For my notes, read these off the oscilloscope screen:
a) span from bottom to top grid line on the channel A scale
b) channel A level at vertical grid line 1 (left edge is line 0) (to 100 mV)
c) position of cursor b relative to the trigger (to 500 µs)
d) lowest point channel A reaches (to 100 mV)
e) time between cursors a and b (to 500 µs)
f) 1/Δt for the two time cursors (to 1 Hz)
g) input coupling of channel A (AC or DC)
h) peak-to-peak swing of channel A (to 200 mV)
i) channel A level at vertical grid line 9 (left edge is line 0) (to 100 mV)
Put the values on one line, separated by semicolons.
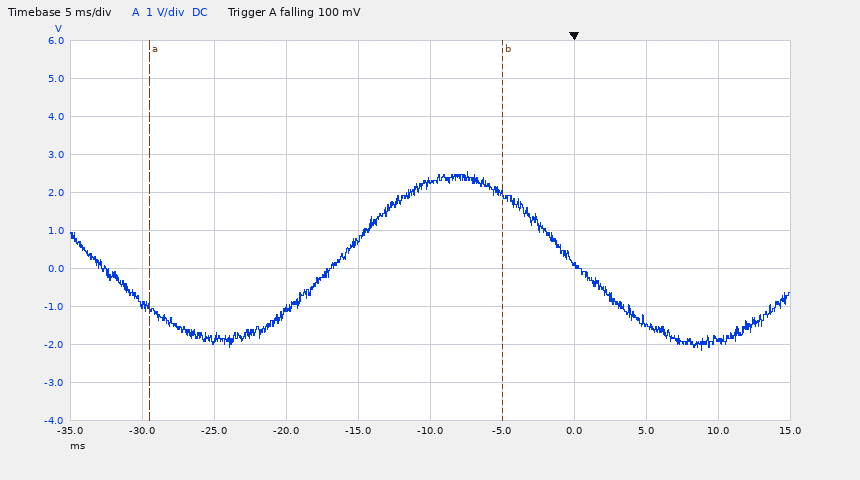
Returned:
10 V; -1.0 V; -5.0 ms; -2.2 V; 24.5 ms; 41 Hz; DC; 4.8 V; -1.9 V
